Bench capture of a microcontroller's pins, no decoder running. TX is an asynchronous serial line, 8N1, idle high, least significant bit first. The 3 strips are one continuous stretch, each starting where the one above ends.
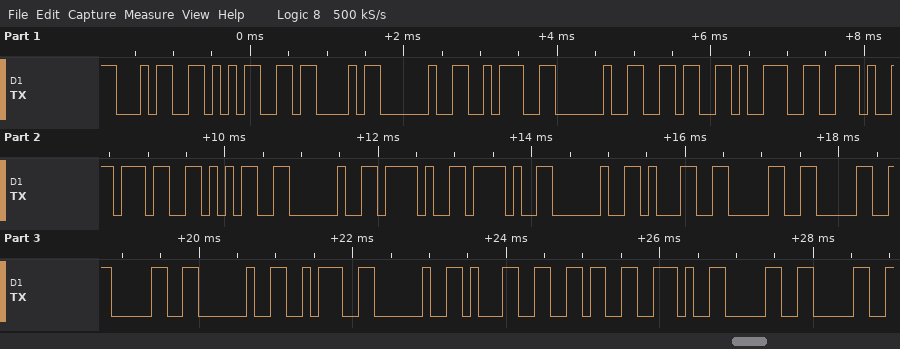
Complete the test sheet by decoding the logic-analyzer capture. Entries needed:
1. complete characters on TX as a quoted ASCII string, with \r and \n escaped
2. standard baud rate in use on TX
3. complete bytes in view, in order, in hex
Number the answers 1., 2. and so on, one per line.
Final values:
1. "45C : 69.75 // 1000 : 16.00"
2. 9600 baud
3. 34 35 43 20 3A 20 36 39 2E 37 35 20 2F 2F 20 31 30 30 30 20 3A 20 31 36 2E 30 30
